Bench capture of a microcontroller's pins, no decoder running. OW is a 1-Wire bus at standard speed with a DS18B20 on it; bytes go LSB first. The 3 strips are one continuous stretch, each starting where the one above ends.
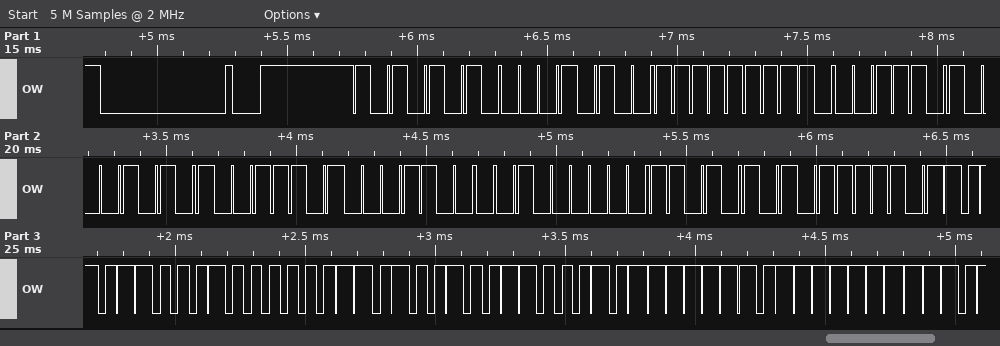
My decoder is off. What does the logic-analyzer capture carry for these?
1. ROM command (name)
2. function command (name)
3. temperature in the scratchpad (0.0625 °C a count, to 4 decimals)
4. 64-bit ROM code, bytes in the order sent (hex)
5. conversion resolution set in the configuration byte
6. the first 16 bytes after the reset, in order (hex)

Match ROM
Read Scratchpad
35.3125 °C
28 FF 71 51 B9 18 02 AB
12 bits
55 28 FF 71 51 B9 18 02 AB BE 35 02 4B 46 7F FF
